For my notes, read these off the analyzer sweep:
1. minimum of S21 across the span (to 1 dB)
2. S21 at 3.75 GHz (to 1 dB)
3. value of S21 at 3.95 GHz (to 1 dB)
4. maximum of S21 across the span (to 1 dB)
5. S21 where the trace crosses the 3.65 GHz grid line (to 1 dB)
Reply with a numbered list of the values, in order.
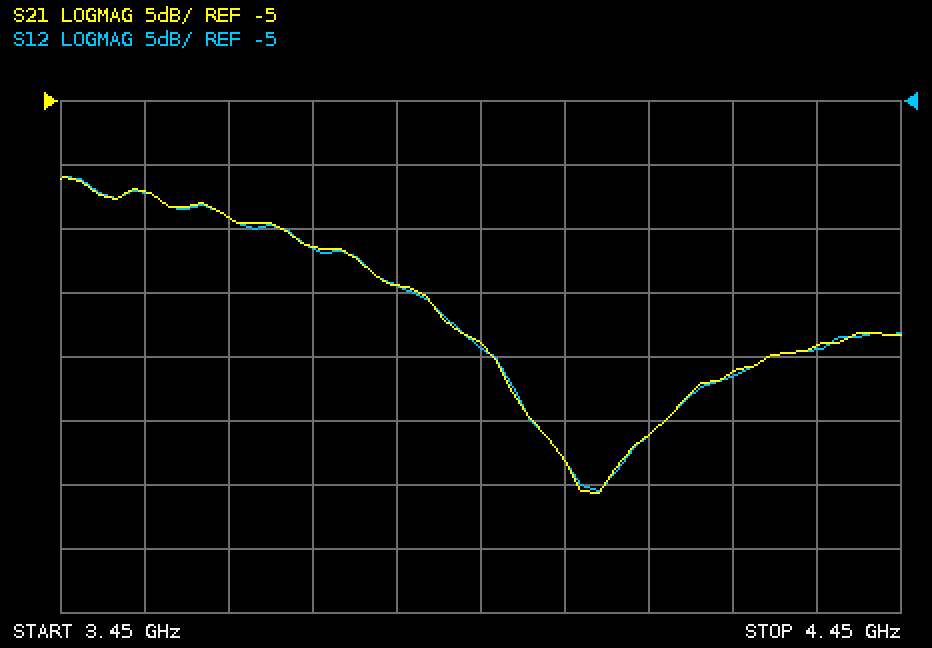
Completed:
1. -36 dB
2. -16 dB
3. -24 dB
4. -11 dB
5. -14 dB
